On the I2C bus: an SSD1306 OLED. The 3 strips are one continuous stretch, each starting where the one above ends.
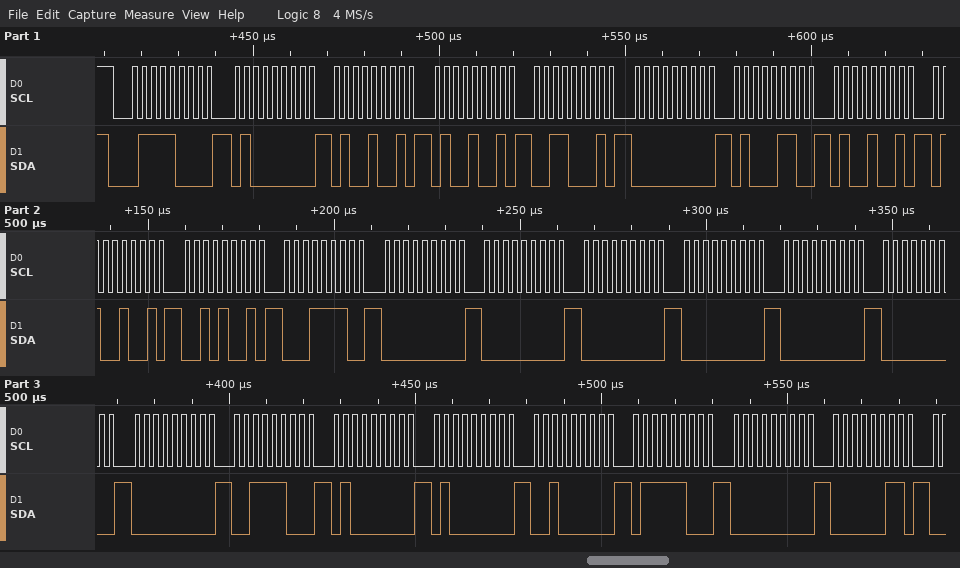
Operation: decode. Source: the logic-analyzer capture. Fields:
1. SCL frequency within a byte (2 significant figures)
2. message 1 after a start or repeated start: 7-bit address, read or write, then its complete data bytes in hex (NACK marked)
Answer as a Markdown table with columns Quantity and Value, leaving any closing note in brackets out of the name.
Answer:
| Quantity | Value |
|---|---|
| SCL frequency within a byte | 400 kHz |
| message 1 after a start or repeated start: 7-bit address, read or write, then its complete data bytes in hex | 0x3C write: 40 49 49 31 00 46 49 49 29 1E 00 00 00 00 00 00 00 3C 40 40 20 7C 00 03 |
